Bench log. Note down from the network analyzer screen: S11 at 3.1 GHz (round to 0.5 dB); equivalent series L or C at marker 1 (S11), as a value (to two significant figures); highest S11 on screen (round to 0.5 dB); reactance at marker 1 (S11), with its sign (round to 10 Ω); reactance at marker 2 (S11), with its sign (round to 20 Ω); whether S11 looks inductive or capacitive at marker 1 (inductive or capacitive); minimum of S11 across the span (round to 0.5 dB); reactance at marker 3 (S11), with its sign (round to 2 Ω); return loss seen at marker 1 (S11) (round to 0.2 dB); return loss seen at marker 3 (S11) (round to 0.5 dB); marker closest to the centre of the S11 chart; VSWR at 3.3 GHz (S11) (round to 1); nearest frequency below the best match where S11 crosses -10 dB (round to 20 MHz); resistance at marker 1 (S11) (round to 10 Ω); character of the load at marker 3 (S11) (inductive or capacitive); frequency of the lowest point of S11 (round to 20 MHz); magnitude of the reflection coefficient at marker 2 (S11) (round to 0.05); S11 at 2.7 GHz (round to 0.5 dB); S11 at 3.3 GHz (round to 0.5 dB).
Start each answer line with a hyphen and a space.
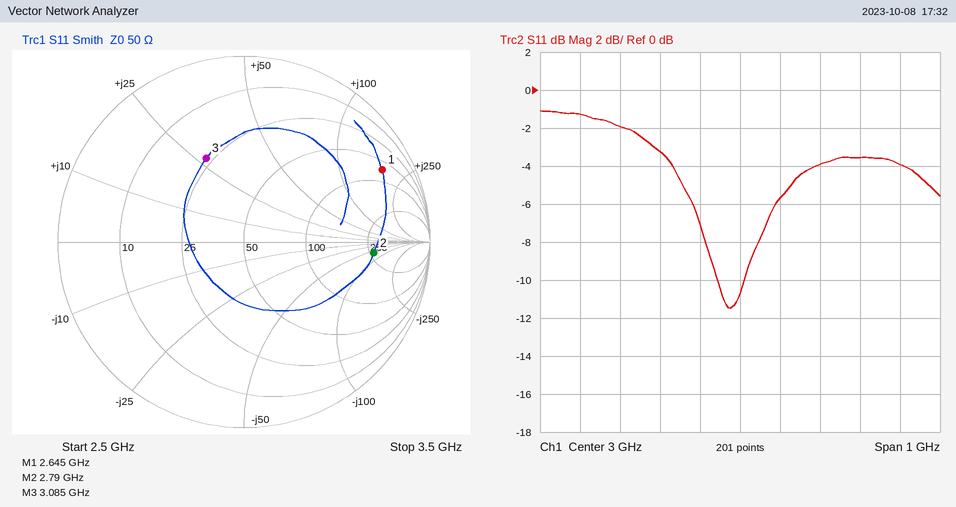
- -5.5 dB
- 11 nH
- -1.0 dB
- +180 Ω
- -60 Ω
- inductive
- -11.5 dB
- +28 Ω
- 1.6 dB
- 6.0 dB
- marker 3
- 5
- 2.94 GHz
- 70 Ω
- inductive
- 2.98 GHz
- 0.70
- -2.0 dB
- -3.5 dB
